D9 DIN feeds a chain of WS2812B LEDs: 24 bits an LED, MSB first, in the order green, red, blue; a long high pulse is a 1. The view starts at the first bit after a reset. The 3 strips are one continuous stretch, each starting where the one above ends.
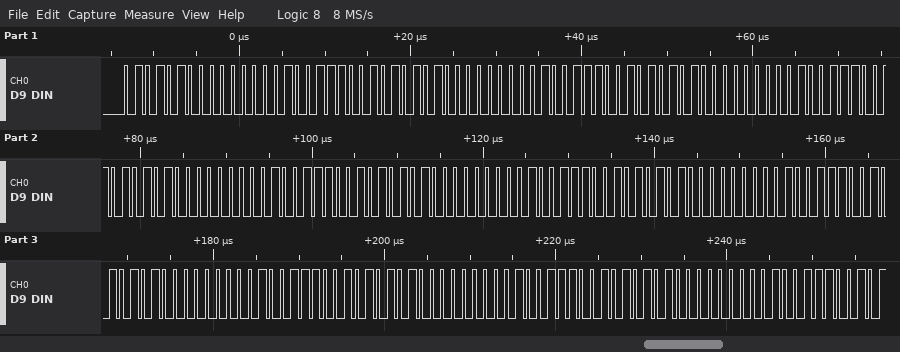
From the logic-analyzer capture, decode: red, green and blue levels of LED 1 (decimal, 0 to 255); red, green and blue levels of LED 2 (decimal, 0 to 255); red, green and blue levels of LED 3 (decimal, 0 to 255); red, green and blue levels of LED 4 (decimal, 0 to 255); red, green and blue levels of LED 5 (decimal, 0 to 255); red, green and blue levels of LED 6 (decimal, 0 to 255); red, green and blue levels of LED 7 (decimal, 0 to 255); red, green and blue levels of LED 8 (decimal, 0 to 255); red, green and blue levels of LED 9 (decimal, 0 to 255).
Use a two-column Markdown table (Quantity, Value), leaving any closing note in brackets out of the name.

| Quantity | Value |
|---|---|
| red, green and blue levels of LED 1 | 1, 84, 57 |
| red, green and blue levels of LED 2 | 1, 84, 57 |
| red, green and blue levels of LED 3 | 1, 84, 57 |
| red, green and blue levels of LED 4 | 1, 84, 57 |
| red, green and blue levels of LED 5 | 1, 84, 57 |
| red, green and blue levels of LED 6 | 1, 84, 57 |
| red, green and blue levels of LED 7 | 1, 84, 57 |
| red, green and blue levels of LED 8 | 1, 84, 57 |
| red, green and blue levels of LED 9 | 1, 84, 57 |
